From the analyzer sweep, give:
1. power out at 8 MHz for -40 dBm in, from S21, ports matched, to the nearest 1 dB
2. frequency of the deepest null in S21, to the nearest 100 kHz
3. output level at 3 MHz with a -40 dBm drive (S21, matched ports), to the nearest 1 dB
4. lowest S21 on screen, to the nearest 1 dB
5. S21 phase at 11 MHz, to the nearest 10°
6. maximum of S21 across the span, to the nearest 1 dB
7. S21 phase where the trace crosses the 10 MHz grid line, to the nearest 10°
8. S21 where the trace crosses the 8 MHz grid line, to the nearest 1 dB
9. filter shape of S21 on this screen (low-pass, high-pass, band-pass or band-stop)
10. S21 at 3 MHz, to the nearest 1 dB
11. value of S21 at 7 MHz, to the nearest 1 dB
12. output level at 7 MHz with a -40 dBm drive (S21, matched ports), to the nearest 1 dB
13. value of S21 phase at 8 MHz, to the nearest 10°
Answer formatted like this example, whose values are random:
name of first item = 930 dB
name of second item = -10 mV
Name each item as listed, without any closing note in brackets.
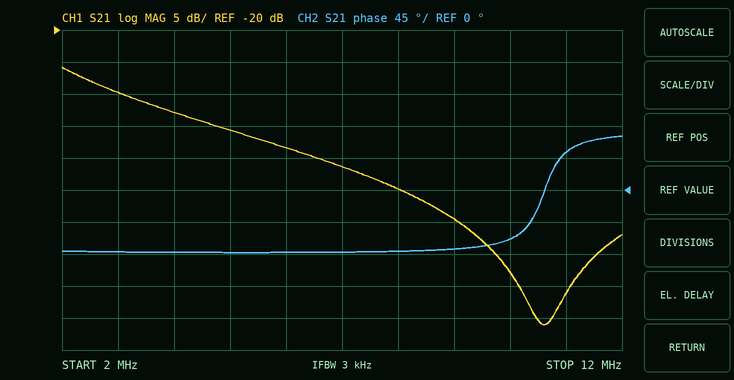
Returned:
power out at 8 MHz for -40 dBm in, from S21, ports matched, to the nearest 1 dB = -85 dBm
frequency of the deepest null in S21, to the nearest 100 kHz = 10.6 MHz
output level at 3 MHz with a -40 dBm drive (S21, matched ports), to the nearest 1 dB = -70 dBm
lowest S21 on screen, to the nearest 1 dB = -66 dB
S21 phase at 11 MHz, to the nearest 10° = 50°
maximum of S21 across the span, to the nearest 1 dB = -26 dB
S21 phase where the trace crosses the 10 MHz grid line, to the nearest 10° = -70°
S21 where the trace crosses the 8 MHz grid line, to the nearest 1 dB = -45 dB
filter shape of S21 on this screen = low-pass
S21 at 3 MHz, to the nearest 1 dB = -30 dB
value of S21 at 7 MHz, to the nearest 1 dB = -41 dB
output level at 7 MHz with a -40 dBm drive (S21, matched ports), to the nearest 1 dB = -81 dBm
value of S21 phase at 8 MHz, to the nearest 10° = -90°
